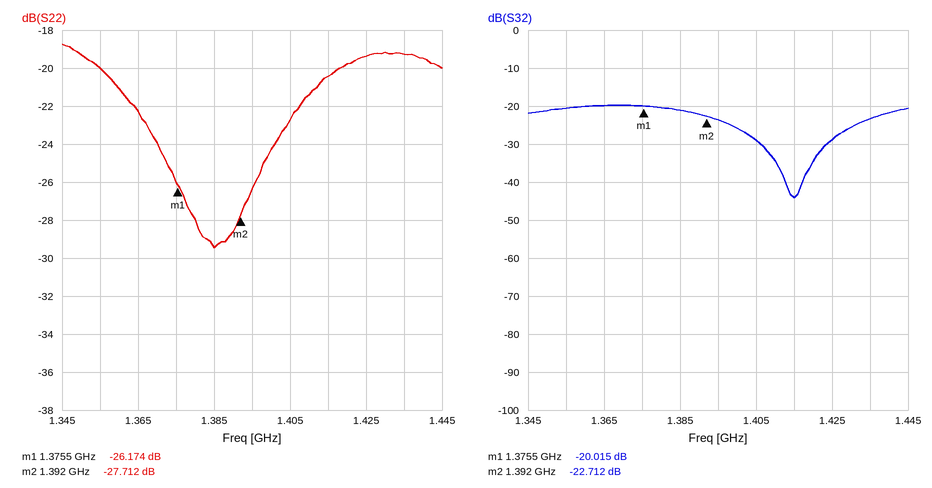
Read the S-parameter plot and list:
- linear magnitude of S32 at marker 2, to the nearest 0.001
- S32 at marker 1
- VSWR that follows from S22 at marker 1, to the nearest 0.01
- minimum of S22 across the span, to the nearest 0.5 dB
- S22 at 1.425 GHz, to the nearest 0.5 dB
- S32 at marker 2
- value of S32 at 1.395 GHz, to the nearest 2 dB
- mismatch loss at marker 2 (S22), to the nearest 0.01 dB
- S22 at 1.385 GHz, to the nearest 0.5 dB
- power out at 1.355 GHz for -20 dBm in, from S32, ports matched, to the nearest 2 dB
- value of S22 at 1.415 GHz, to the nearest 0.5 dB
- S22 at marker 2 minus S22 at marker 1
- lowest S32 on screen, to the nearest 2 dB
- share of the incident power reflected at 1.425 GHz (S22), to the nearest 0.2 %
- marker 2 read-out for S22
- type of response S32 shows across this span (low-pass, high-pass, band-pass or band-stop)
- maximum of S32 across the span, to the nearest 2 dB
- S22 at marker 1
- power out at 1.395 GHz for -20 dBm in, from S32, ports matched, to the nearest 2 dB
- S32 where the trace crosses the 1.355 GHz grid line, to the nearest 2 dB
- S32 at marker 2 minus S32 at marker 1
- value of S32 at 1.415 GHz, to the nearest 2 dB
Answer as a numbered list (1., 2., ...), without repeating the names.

1. 0.073
2. -20.015 dB
3. 1.10
4. -29.5 dB
5. -19.5 dB
6. -22.712 dB
7. -24 dB
8. 0.01 dB
9. -29.5 dB
10. -40 dBm
11. -20.5 dB
12. -1.538 dB
13. -44 dB
14. 1.2 %
15. -27.712 dB
16. band-stop
17. -20 dB
18. -26.174 dB
19. -44 dBm
20. -20 dB
21. -2.697 dB
22. -44 dB
